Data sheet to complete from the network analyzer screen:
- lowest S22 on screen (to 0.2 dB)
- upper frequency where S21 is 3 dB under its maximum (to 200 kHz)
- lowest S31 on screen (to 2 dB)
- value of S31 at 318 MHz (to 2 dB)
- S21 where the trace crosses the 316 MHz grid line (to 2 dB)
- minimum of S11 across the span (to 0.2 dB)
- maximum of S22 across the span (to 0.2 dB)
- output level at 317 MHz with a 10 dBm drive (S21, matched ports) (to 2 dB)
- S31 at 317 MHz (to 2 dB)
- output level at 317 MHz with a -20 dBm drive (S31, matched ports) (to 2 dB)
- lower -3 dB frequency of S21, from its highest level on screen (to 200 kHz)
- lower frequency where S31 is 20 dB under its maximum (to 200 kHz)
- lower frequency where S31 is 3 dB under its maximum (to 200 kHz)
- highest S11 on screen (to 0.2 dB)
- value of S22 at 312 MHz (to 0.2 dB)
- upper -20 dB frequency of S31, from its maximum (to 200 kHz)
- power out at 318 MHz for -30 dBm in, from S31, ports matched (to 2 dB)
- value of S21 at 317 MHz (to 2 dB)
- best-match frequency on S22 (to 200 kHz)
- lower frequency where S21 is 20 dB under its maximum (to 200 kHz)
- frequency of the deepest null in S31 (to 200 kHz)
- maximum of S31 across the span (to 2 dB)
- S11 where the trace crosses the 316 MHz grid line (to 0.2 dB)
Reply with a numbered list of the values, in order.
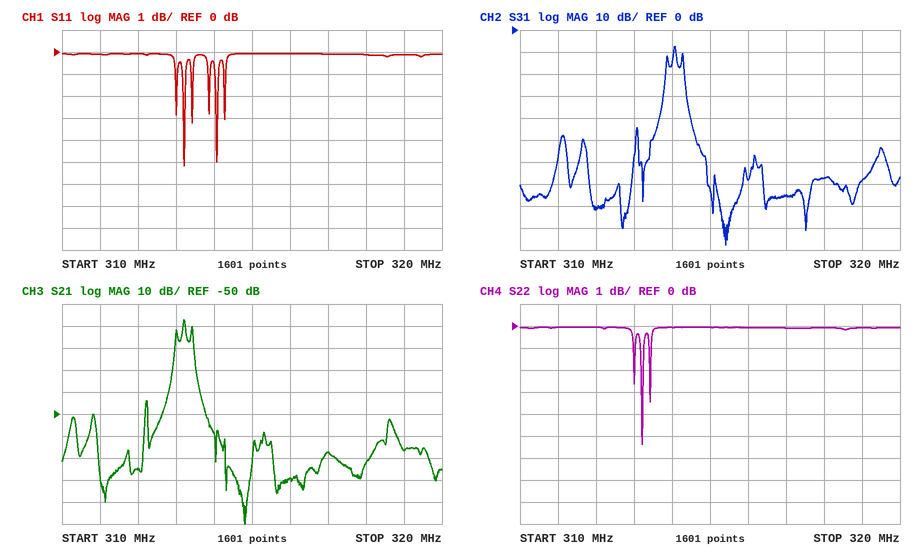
1. -5.4 dB
2. 313.2 MHz
3. -98 dB
4. -68 dB
5. -80 dB
6. -5.2 dB
7. 0.0 dB
8. -58 dBm
9. -76 dB
10. -96 dBm
11. 313.2 MHz
12. 313.8 MHz
13. 314.0 MHz
14. 0.0 dB
15. 0.0 dB
16. 314.4 MHz
17. -98 dBm
18. -68 dB
19. 313.2 MHz
20. 313.0 MHz
21. 315.4 MHz
22. -8 dB
23. 0.0 dB
